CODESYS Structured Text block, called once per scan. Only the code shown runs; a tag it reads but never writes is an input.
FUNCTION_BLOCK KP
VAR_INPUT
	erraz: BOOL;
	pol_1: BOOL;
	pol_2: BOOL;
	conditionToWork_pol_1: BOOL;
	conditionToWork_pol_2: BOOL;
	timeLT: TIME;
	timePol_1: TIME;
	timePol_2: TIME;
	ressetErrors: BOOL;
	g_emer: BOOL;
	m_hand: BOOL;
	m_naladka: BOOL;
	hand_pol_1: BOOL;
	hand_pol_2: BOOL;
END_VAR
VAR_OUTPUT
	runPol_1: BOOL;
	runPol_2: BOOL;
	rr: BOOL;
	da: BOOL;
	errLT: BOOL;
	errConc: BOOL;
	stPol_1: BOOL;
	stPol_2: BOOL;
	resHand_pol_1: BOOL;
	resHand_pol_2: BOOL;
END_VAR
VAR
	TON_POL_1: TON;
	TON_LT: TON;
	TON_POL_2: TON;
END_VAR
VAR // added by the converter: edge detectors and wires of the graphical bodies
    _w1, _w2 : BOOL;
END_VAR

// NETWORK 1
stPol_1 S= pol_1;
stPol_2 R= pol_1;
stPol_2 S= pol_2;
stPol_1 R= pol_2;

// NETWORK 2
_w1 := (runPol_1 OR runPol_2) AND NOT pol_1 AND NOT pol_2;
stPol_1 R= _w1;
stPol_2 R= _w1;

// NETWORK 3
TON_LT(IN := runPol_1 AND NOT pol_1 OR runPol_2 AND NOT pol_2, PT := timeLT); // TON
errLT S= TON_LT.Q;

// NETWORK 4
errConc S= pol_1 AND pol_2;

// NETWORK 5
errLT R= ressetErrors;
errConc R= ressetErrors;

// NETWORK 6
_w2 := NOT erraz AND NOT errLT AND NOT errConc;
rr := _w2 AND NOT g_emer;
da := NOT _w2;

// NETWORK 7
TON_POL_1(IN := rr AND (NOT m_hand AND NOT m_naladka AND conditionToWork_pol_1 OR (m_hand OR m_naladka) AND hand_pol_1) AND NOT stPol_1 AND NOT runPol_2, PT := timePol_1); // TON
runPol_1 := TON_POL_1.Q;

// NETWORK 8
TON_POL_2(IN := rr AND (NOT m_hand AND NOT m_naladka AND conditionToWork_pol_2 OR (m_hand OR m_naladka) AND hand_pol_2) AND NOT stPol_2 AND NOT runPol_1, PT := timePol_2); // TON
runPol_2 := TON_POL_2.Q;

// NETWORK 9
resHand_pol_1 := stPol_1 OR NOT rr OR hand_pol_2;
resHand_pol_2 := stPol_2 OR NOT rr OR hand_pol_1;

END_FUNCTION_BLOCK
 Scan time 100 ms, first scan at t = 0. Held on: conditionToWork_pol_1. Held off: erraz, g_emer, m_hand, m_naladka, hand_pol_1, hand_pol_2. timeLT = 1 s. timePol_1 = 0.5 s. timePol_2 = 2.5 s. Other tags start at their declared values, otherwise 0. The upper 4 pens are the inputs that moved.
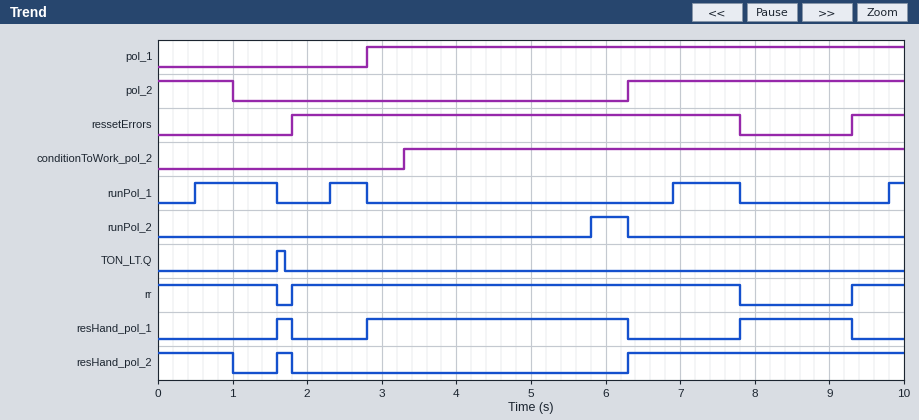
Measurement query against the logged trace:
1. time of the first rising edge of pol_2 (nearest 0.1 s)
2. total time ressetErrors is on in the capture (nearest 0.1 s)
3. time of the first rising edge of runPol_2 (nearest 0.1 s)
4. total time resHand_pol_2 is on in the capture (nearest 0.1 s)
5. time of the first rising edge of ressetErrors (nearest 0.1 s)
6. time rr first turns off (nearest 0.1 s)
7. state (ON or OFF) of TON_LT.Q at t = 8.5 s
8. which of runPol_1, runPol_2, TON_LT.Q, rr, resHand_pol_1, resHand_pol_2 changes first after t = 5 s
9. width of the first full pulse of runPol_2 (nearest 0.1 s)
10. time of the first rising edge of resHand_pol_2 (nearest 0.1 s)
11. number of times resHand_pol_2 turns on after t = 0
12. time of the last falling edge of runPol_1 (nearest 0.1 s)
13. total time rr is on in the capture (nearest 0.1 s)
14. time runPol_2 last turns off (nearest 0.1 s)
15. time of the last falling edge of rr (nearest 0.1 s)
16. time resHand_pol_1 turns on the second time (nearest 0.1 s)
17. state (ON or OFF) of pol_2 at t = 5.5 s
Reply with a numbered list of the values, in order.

1. 6.3 s
2. 6.7 s
3. 5.8 s
4. 4.9 s
5. 1.8 s
6. 1.6 s
7. OFF
8. runPol_2
9. 0.5 s
10. 1.6 s
11. 2
12. 7.8 s
13. 8.3 s
14. 6.3 s
15. 7.8 s
16. 2.8 s
17. OFF
